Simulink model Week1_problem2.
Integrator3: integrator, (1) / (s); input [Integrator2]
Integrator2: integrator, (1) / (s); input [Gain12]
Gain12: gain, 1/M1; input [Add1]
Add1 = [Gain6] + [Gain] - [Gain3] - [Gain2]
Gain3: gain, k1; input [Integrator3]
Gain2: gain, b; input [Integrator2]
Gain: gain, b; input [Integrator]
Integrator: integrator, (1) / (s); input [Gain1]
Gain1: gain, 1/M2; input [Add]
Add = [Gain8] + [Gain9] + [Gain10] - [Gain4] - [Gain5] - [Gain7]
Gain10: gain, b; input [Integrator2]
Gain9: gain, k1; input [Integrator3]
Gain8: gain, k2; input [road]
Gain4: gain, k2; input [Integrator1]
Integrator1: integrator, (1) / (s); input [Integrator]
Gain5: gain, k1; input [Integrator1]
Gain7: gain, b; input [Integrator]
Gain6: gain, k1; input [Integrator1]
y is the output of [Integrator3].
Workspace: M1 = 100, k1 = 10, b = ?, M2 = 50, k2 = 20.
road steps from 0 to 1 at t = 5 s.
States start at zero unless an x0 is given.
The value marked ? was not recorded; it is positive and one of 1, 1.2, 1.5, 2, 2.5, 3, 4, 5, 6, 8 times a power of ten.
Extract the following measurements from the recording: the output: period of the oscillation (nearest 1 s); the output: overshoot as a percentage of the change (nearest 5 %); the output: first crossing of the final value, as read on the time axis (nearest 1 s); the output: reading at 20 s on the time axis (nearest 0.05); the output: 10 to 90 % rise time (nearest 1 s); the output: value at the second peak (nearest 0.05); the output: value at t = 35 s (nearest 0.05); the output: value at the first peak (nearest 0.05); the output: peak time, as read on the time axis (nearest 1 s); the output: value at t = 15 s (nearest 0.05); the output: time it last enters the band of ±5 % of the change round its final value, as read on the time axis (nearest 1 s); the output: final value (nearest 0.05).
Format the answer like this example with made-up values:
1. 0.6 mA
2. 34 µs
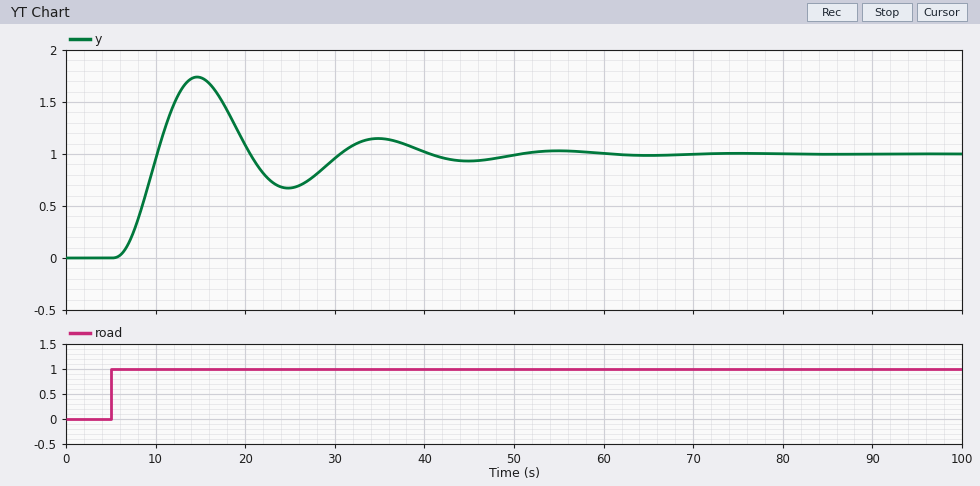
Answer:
1. 20 s
2. 75 %
3. 10 s
4. 1.10
5. 3 s
6. 1.15
7. 1.15
8. 1.75
9. 15 s
10. 1.75
11. 47 s
12. 1.00
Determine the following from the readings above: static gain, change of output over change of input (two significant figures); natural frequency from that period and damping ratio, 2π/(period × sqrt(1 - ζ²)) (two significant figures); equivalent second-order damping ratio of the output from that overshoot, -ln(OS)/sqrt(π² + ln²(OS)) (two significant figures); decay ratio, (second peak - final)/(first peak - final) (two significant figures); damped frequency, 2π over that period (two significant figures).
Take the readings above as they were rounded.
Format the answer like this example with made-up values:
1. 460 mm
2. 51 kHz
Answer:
1. 1.0
2. 0.32 rad/s
3. 0.091
4. 0.20
5. 0.31 rad/s
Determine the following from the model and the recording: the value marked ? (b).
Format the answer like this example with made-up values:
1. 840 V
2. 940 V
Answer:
1. 50
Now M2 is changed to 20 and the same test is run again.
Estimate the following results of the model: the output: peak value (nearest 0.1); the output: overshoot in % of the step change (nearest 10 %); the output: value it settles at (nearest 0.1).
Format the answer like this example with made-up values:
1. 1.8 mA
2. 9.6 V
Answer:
1. 1.6
2. 60 %
3. 1.0
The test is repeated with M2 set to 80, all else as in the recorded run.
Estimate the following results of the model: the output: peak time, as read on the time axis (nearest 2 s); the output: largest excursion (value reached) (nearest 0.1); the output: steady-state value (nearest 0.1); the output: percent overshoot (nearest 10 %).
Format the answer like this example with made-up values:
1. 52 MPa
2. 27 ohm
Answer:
1. 16 s
2. 1.8
3. 1.0
4. 80 %
